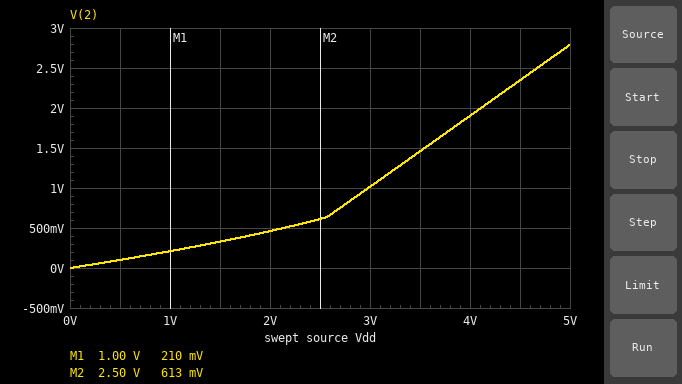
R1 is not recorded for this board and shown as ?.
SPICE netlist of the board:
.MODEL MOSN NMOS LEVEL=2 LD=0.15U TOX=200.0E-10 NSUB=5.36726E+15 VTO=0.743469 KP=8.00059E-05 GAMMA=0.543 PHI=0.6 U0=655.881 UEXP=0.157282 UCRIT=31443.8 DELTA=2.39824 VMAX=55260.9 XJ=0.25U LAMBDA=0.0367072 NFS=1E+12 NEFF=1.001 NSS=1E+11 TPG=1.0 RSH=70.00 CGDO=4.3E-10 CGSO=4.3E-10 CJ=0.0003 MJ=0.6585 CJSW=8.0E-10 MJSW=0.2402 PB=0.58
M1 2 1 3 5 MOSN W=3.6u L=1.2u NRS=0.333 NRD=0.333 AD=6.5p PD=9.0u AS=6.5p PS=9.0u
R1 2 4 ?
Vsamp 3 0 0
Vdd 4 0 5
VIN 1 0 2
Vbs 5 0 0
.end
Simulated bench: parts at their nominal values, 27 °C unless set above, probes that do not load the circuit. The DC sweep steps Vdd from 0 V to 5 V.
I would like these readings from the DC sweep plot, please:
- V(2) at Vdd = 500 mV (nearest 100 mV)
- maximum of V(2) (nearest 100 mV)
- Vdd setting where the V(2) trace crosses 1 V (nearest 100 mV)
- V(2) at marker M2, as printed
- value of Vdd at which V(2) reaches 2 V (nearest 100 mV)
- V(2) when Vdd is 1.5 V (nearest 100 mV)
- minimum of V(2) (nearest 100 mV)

100 mV
2.8 V
3.0 V
613 mV
4.1 V
300 mV
0 V
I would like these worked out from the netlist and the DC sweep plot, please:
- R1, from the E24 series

13 kΩ
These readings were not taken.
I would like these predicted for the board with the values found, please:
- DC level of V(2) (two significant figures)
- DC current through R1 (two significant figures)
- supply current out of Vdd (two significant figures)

2.8 V
170 µA
170 µA
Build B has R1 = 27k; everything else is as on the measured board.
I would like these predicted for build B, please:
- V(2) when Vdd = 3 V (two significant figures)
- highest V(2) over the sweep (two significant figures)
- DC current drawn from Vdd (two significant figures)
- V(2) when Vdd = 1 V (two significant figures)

360 mV
910 mV
150 µA
110 mV
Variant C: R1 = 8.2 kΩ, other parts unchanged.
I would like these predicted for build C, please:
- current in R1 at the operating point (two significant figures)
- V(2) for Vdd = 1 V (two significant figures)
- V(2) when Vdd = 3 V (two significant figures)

180 µA
310 mV
1.7 V
